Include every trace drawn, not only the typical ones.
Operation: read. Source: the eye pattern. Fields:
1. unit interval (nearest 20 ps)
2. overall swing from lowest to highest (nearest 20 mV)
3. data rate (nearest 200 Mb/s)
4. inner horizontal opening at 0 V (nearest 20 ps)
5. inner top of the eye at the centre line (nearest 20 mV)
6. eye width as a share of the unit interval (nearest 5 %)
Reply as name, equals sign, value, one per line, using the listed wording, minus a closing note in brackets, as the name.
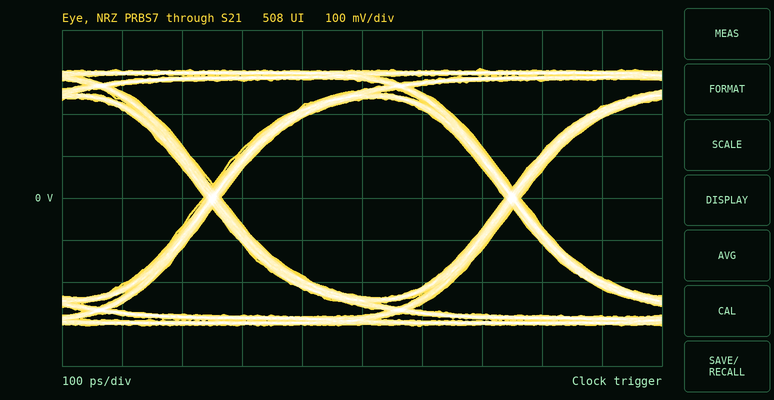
unit interval = 500 ps
overall swing from lowest to highest = 620 mV
data rate = 2.0 Gb/s
inner horizontal opening at 0 V = 480 ps
inner top of the eye at the centre line = 240 mV
eye width as a share of the unit interval = 95 %
